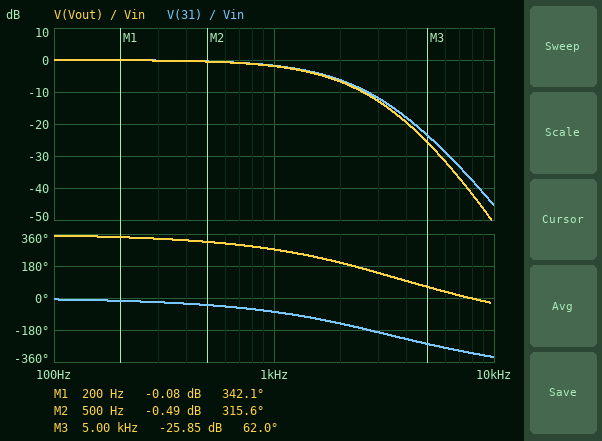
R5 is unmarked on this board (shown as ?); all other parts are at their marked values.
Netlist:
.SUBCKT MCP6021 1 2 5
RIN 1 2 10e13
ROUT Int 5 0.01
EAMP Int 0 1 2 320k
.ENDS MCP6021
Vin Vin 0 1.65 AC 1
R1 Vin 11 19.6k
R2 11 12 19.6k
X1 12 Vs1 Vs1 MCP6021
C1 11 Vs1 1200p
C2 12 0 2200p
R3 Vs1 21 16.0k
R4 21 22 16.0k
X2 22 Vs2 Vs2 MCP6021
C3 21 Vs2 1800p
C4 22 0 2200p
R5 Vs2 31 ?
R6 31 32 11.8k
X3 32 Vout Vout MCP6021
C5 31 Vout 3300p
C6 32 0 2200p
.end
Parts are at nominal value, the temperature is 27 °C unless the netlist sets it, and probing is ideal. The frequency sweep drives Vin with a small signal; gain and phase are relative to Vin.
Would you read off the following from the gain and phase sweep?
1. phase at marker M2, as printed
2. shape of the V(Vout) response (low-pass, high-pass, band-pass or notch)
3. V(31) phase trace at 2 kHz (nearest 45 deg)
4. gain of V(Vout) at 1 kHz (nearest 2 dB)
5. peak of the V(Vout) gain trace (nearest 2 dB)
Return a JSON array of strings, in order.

["315.6 deg", "low-pass", "-135 deg", "-2 dB", "0 dB"]
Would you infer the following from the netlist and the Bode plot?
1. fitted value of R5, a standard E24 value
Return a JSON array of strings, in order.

["30 kΩ"]
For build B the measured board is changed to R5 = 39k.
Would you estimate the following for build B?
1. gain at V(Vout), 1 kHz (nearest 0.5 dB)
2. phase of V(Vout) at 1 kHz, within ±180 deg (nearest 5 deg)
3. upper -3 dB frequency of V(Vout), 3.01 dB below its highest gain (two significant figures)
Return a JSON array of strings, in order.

["-2.5 dB", "-95 deg", "1.2 kHz"]
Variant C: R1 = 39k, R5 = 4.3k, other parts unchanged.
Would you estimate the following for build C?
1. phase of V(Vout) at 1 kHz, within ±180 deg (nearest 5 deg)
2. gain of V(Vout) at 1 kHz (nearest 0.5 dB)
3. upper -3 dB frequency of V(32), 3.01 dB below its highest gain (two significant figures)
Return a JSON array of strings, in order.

["-80 deg", "-2.5 dB", "1.2 kHz"]
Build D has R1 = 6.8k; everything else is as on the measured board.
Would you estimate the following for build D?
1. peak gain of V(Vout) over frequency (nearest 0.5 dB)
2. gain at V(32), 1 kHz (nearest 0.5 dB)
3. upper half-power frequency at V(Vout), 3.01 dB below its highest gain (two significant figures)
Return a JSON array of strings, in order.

["0 dB", "-1.5 dB", "1.4 kHz"]
